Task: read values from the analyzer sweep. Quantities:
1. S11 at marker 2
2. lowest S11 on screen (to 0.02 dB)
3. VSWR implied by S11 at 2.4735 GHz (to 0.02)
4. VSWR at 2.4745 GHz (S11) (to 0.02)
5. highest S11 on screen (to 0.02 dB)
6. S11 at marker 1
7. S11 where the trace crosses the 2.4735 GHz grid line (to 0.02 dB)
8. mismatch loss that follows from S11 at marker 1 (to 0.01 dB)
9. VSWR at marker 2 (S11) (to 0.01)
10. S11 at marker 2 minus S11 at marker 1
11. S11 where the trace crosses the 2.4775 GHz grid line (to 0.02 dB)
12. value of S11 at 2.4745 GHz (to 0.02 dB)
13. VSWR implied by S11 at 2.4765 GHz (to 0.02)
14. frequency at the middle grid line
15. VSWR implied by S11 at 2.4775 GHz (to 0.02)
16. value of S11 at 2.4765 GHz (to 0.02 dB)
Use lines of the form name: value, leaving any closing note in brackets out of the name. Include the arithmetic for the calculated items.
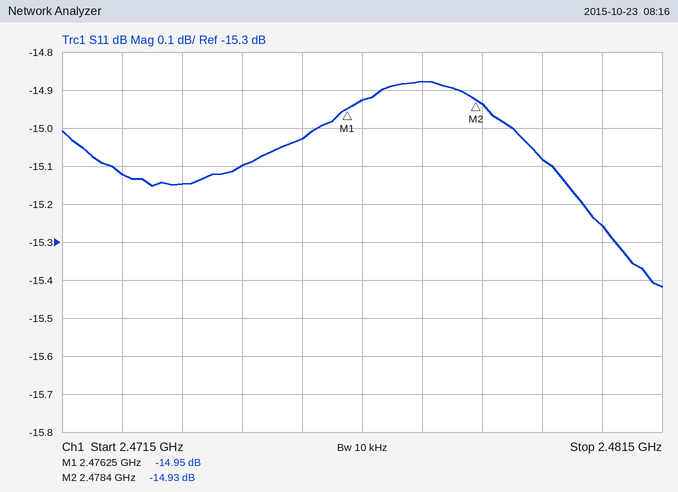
S11 at marker 2: -14.93 dB
lowest S11 on screen: -15.42 dB
VSWR implied by S11 at 2.4735 GHz: |Γ| = 10^(-15.14/20) = 0.1750; VSWR = (1 + 0.1750)/(1 − 0.1750) ≈ 1.42
VSWR at 2.4745 GHz (S11): |Γ| = 10^(-15.1/20) = 0.1758; VSWR = (1 + 0.1758)/(1 − 0.1758) ≈ 1.43, so 1.42 to the nearest 0.02
highest S11 on screen: -14.88 dB
S11 at marker 1: -14.95 dB
S11 where the trace crosses the 2.4735 GHz grid line: -15.14 dB
mismatch loss that follows from S11 at marker 1: −10 log10(1 − 10^(-14.95/10)) ≈ 0.14 dB
VSWR at marker 2 (S11): (1 + 0.1793)/(1 − 0.1793) ≈ 1.44
S11 at marker 2 minus S11 at marker 1: -14.93 − (-14.95) = 0.02 dB
S11 where the trace crosses the 2.4775 GHz grid line: -14.88 dB
value of S11 at 2.4745 GHz: -15.10 dB
VSWR implied by S11 at 2.4765 GHz: |Γ| = 10^(-14.92/20) = 0.1795; VSWR = (1 + 0.1795)/(1 − 0.1795) ≈ 1.44
frequency at the middle grid line: 2.4765 GHz
VSWR implied by S11 at 2.4775 GHz: |Γ| = 10^(-14.88/20) = 0.1803; VSWR = (1 + 0.1803)/(1 − 0.1803) ≈ 1.44
value of S11 at 2.4765 GHz: -14.92 dB
